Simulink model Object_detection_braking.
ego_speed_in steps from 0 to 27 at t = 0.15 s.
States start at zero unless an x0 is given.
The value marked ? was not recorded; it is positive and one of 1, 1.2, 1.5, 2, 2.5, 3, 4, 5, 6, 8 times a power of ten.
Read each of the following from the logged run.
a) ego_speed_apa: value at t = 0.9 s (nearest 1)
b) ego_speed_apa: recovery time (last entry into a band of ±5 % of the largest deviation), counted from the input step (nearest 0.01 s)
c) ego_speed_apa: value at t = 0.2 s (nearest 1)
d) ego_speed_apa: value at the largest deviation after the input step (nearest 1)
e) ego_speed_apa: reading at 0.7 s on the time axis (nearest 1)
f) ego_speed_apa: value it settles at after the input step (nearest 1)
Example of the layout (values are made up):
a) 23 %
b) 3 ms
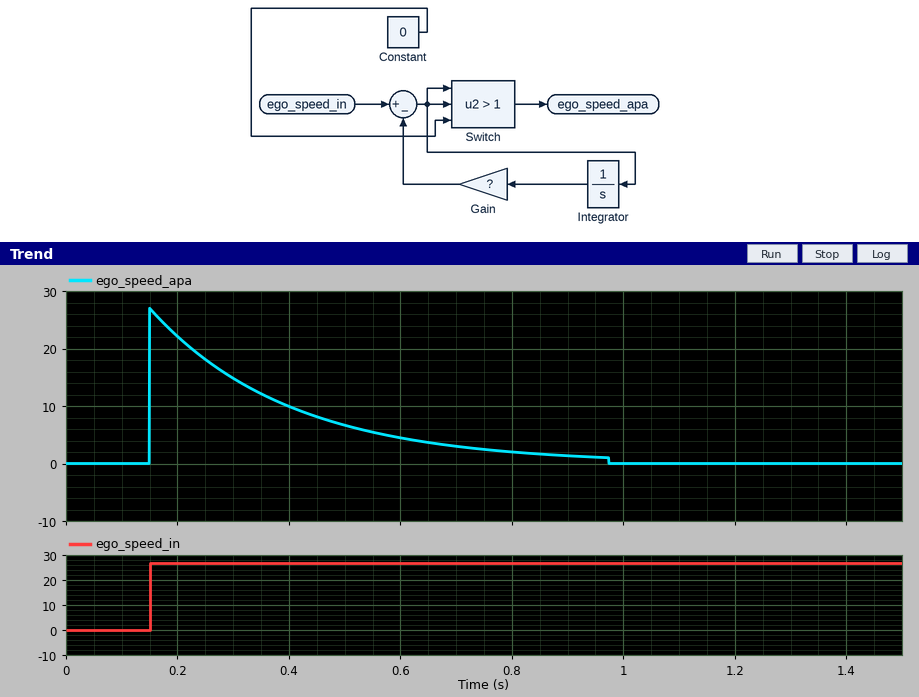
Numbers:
a) 1
b) 0.75 s
c) 22
d) 27
e) 3
f) 0
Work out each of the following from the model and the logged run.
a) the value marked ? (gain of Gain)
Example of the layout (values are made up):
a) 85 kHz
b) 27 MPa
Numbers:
a) 4
